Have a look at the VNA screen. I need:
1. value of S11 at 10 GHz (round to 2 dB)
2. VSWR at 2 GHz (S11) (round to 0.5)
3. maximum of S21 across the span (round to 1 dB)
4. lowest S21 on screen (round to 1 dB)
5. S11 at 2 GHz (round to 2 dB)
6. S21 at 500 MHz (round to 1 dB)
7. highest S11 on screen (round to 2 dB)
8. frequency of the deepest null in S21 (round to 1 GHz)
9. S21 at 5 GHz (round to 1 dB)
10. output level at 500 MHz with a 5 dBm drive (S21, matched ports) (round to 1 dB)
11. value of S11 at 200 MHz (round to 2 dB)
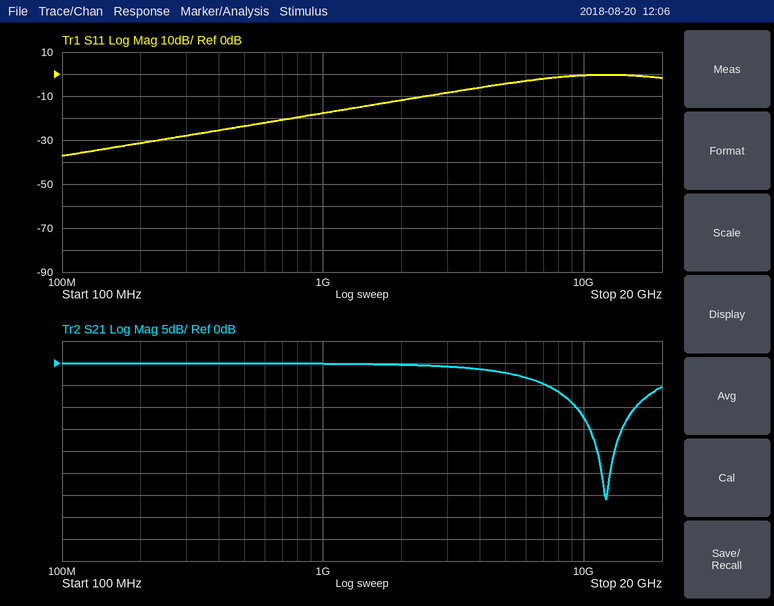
0 dB
1.5
0 dB
-31 dB
-12 dB
0 dB
0 dB
12 GHz
-2 dB
5 dBm
-32 dB
